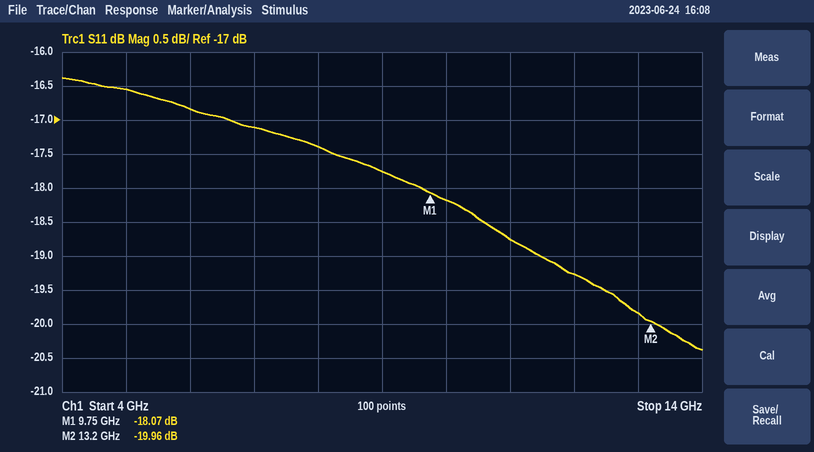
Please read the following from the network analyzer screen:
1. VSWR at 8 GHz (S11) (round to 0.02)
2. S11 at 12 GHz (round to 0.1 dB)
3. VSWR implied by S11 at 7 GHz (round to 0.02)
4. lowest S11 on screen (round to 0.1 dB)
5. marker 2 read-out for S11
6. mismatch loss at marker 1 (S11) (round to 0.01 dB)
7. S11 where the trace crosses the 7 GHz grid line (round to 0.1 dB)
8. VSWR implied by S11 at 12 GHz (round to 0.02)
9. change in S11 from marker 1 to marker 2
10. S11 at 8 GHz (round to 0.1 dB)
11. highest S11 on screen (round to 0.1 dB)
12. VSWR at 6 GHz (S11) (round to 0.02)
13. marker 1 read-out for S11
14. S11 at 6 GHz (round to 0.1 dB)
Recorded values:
1.32
-19.3 dB
1.32
-20.4 dB
-19.96 dB
0.07 dB
-17.1 dB
1.24
-1.89 dB
-17.4 dB
-16.4 dB
1.34
-18.07 dB
-16.8 dB
